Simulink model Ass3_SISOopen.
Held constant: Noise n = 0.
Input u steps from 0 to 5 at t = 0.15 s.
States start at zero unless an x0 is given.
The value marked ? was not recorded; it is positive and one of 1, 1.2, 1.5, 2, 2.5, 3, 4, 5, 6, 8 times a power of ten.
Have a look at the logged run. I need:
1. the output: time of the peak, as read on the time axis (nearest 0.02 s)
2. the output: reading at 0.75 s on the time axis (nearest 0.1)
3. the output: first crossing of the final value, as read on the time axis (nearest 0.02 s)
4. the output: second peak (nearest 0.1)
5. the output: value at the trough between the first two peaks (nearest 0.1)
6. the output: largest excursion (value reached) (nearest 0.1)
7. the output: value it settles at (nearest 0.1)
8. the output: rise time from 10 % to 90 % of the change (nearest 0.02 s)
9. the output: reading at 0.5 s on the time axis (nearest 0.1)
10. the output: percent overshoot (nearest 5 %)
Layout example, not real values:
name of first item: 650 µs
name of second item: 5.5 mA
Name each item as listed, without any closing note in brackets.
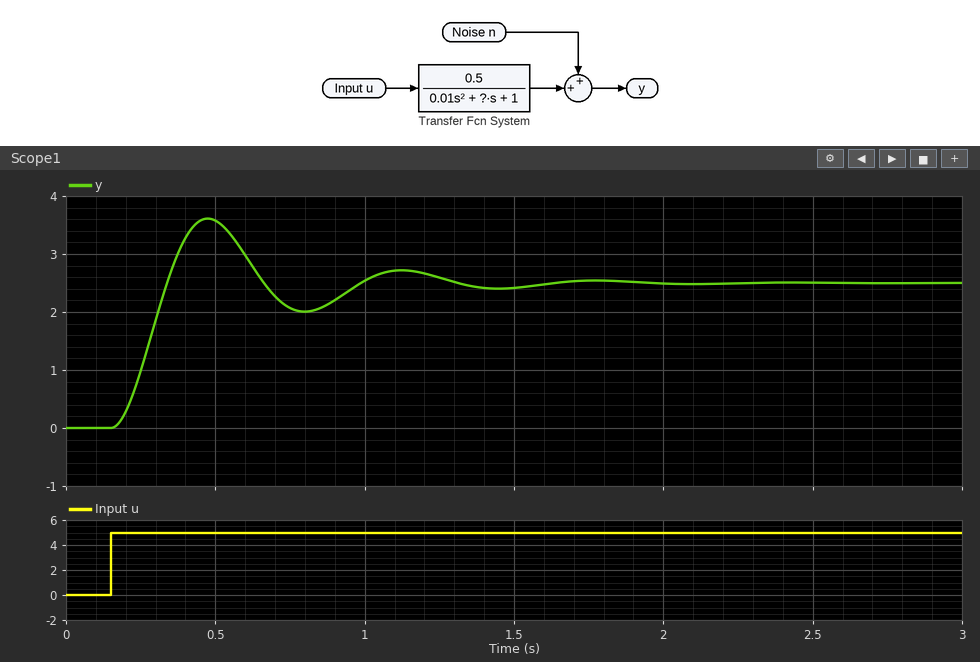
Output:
the output: time of the peak, as read on the time axis: 0.48 s
the output: reading at 0.75 s on the time axis: 2.1
the output: first crossing of the final value, as read on the time axis: 0.34 s
the output: second peak: 2.7
the output: value at the trough between the first two peaks: 2.0
the output: largest excursion (value reached): 3.6
the output: value it settles at: 2.5
the output: rise time from 10 % to 90 % of the change: 0.12 s
the output: reading at 0.5 s on the time axis: 3.6
the output: percent overshoot: 45 %
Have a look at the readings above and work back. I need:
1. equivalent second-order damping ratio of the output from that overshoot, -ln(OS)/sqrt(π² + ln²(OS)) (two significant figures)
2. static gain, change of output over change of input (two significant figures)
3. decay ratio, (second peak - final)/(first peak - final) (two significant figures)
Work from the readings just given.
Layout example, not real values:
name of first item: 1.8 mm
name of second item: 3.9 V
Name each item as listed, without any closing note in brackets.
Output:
equivalent second-order damping ratio of the output from that overshoot, -ln(OS)/sqrt(π² + ln²(OS)): 0.25
static gain, change of output over change of input: 0.50
decay ratio, (second peak - final)/(first peak - final): 0.18
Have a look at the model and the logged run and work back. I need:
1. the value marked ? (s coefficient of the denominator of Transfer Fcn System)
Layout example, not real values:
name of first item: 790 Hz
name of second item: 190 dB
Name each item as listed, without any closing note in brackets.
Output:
the value marked ?: 0.05
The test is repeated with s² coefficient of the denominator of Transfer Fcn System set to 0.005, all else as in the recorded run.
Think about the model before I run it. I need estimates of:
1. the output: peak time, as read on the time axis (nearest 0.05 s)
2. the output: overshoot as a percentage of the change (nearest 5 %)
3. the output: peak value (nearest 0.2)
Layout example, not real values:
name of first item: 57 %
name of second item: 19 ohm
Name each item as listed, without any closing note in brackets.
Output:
the output: peak time, as read on the time axis: 0.40 s
the output: overshoot as a percentage of the change: 30 %
the output: peak value: 3.2
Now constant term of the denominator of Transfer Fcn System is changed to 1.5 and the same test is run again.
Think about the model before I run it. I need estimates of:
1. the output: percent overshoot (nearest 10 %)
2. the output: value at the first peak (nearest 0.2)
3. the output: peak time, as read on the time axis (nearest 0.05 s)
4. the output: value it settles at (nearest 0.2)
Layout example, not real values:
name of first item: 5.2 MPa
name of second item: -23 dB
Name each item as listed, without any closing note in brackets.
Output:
the output: percent overshoot: 50 %
the output: value at the first peak: 2.6
the output: peak time, as read on the time axis: 0.40 s
the output: value it settles at: 1.6
